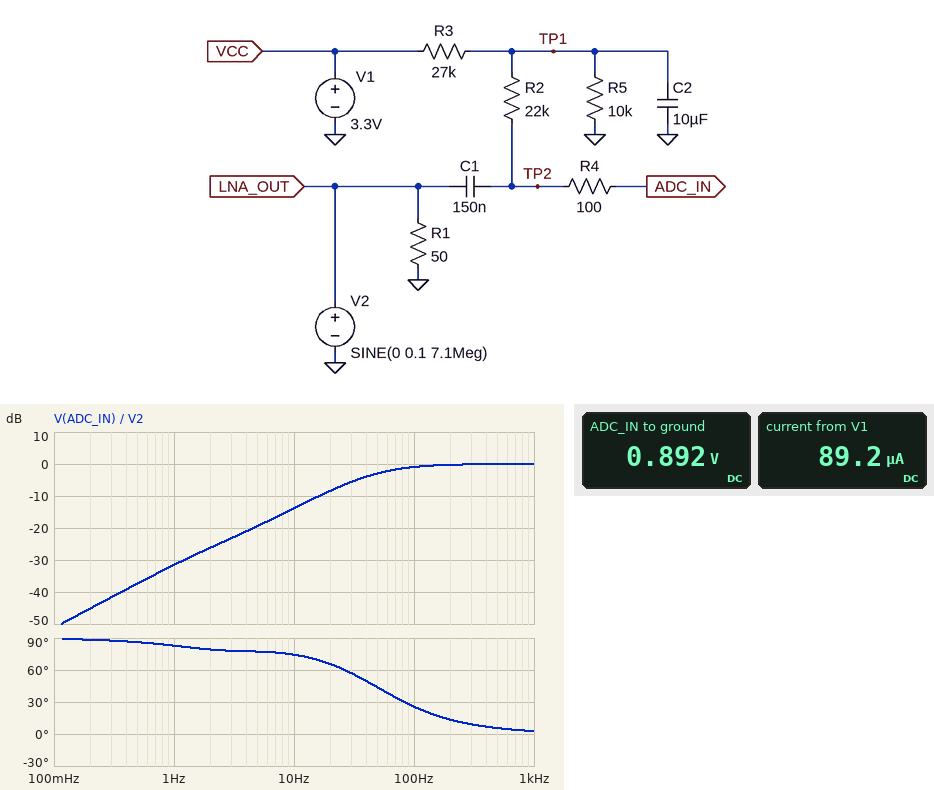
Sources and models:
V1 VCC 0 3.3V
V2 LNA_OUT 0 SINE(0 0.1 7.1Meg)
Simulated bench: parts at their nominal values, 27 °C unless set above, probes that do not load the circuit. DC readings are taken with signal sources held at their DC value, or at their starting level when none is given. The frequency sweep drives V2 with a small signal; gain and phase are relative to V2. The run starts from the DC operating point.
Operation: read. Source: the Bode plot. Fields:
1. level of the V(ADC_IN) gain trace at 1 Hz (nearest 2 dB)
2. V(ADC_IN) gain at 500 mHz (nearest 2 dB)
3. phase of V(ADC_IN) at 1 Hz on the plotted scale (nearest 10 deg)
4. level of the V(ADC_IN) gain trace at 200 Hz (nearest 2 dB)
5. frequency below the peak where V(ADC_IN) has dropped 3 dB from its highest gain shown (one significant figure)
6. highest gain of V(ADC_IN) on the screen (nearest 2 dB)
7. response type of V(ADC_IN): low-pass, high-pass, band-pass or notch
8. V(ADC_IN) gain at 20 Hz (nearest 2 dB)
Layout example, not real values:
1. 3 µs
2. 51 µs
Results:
1. -32 dB
2. -38 dB
3. 80 deg
4. 0 dB
5. 50 Hz
6. 0 dB
7. high-pass
8. -8 dB
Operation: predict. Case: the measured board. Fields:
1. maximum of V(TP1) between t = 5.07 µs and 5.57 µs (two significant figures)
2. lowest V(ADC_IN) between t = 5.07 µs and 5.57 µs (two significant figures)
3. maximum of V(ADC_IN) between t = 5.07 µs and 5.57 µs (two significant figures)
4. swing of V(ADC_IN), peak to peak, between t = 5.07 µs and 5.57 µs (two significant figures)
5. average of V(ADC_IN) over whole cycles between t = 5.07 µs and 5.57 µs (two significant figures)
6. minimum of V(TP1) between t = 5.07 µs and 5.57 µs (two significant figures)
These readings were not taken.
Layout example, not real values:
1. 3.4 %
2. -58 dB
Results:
1. 890 mV
2. 790 mV
3. 990 mV
4. 200 mV
5. 890 mV
6. 890 mV
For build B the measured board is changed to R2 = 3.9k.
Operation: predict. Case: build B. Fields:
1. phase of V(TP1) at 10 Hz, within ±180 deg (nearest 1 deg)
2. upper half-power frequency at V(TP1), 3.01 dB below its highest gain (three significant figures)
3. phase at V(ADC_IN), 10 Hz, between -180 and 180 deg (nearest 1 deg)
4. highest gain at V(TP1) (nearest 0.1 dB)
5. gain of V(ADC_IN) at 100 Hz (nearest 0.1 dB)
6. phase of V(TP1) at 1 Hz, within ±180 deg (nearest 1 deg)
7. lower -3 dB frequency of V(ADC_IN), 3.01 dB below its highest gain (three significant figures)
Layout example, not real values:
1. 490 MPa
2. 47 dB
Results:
1. 10 deg
2. 280 Hz
3. 68 deg
4. -36.7 dB
5. -9.3 dB
6. 65 deg
7. 276 Hz
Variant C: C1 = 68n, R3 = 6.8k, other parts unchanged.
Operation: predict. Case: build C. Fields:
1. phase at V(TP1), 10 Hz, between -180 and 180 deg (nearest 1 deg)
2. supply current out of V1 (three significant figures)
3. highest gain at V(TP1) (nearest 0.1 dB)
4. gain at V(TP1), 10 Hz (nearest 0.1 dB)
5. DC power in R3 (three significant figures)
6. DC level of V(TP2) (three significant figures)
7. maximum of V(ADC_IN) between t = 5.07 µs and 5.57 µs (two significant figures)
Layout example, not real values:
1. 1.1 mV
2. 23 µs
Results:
1. 16 deg
2. 196 µA
3. -43.7 dB
4. -44.1 dB
5. 262 µW
6. 1.96 V
7. 2.1 V
